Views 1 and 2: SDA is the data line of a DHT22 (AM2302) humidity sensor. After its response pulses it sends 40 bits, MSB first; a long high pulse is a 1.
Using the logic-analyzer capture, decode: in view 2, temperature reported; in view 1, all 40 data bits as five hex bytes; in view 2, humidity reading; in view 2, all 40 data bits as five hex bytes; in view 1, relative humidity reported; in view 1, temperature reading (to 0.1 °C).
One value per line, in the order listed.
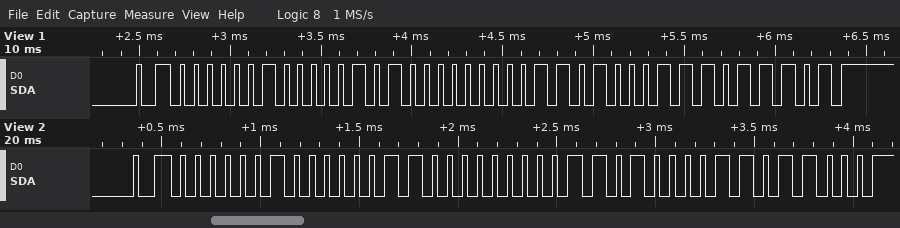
20.8 °C
02 0A 00 D1 DD
51.8 %
02 06 00 D0 D8
52.2 %
20.9 °C
